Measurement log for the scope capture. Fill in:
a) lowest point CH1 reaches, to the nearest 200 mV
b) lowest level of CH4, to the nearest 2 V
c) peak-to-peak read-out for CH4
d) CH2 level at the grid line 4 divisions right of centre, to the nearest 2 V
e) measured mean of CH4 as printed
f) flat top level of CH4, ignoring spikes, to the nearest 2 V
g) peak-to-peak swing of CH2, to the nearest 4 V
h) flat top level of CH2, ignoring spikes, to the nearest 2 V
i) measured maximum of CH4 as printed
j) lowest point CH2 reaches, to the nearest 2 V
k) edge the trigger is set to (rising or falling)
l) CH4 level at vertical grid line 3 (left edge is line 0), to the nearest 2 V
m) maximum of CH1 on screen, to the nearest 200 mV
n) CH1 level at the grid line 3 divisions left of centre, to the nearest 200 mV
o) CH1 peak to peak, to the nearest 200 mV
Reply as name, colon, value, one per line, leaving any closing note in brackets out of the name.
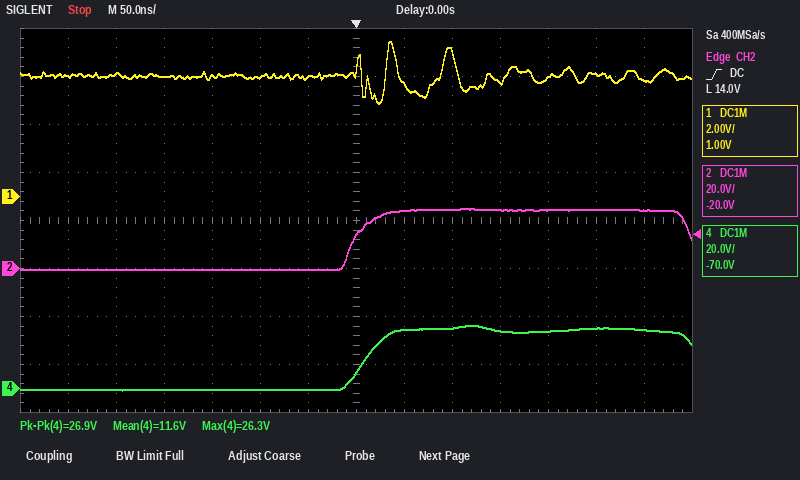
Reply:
lowest point CH1 reaches, to the nearest 200 mV: 3.8 V
lowest level of CH4, to the nearest 2 V: 0 V
peak-to-peak read-out for CH4: 26.9 V
CH2 level at the grid line 4 divisions right of centre, to the nearest 2 V: 24 V
measured mean of CH4 as printed: 11.6 V
flat top level of CH4, ignoring spikes, to the nearest 2 V: 24 V
peak-to-peak swing of CH2, to the nearest 4 V: 24 V
flat top level of CH2, ignoring spikes, to the nearest 2 V: 24 V
measured maximum of CH4 as printed: 26.3 V
lowest point CH2 reaches, to the nearest 2 V: 0 V
edge the trigger is set to: rising
CH4 level at vertical grid line 3 (left edge is line 0), to the nearest 2 V: 0 V
maximum of CH1 on screen, to the nearest 200 mV: 6.4 V
CH1 level at the grid line 3 divisions left of centre, to the nearest 200 mV: 5.0 V
CH1 peak to peak, to the nearest 200 mV: 2.6 V
